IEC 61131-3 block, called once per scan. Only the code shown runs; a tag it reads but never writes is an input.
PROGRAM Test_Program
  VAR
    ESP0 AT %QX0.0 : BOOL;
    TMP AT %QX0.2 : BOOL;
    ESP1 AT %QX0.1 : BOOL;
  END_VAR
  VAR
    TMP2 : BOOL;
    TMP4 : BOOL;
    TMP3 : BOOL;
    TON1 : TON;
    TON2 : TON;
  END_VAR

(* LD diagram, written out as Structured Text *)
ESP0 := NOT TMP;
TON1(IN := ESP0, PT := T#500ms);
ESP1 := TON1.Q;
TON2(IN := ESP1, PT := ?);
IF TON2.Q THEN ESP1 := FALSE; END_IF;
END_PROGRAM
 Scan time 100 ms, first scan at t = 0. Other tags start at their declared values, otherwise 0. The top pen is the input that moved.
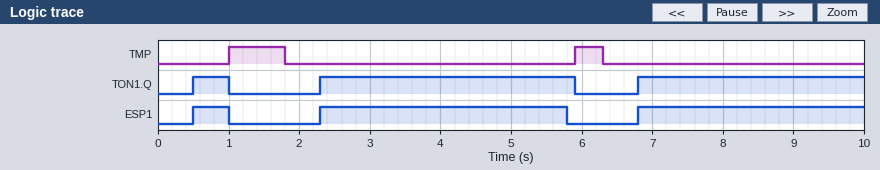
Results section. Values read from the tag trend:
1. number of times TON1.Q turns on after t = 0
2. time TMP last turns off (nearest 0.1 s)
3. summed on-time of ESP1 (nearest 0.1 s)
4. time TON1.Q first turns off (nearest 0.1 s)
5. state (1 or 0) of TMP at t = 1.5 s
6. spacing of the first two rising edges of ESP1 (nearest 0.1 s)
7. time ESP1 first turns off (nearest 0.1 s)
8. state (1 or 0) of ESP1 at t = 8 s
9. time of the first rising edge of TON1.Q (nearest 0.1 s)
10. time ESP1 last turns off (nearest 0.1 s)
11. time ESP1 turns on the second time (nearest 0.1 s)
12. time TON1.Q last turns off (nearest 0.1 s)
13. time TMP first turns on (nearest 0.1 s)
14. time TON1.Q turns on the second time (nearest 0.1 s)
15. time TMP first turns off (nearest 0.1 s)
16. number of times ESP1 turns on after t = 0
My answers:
3
6.3 s
7.2 s
1.0 s
1
1.8 s
1.0 s
1
0.5 s
5.8 s
2.3 s
5.9 s
1.0 s
2.3 s
1.8 s
3
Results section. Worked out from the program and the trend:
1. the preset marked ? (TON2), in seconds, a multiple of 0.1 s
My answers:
3.5 s
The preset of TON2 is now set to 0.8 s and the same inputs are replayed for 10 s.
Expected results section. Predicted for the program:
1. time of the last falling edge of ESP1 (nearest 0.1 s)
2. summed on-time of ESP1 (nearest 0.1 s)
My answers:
7.6 s
2.1 s
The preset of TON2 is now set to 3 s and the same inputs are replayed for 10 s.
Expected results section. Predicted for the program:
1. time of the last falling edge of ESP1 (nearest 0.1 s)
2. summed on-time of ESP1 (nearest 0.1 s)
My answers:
9.8 s
6.5 s
